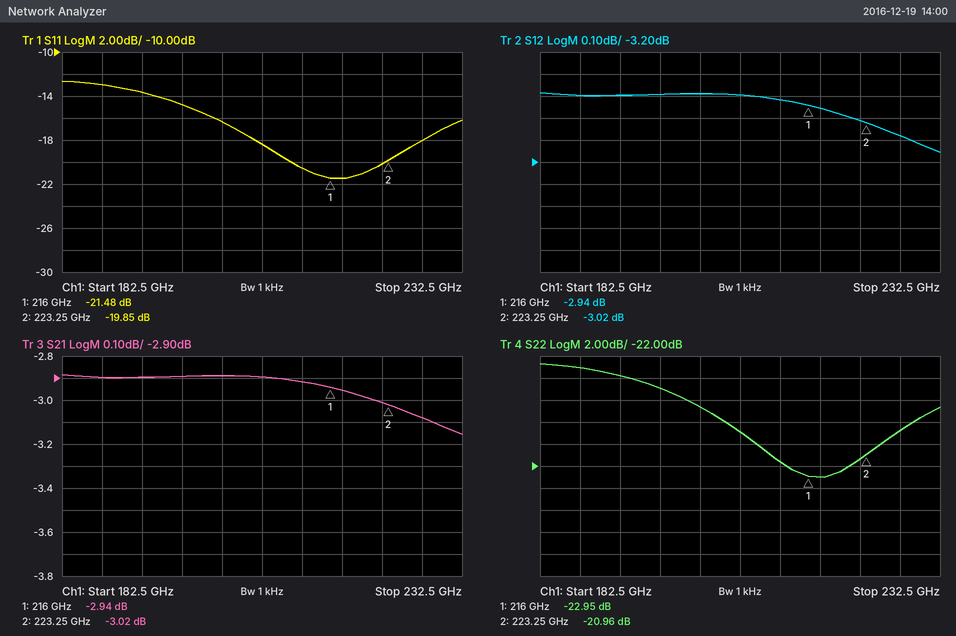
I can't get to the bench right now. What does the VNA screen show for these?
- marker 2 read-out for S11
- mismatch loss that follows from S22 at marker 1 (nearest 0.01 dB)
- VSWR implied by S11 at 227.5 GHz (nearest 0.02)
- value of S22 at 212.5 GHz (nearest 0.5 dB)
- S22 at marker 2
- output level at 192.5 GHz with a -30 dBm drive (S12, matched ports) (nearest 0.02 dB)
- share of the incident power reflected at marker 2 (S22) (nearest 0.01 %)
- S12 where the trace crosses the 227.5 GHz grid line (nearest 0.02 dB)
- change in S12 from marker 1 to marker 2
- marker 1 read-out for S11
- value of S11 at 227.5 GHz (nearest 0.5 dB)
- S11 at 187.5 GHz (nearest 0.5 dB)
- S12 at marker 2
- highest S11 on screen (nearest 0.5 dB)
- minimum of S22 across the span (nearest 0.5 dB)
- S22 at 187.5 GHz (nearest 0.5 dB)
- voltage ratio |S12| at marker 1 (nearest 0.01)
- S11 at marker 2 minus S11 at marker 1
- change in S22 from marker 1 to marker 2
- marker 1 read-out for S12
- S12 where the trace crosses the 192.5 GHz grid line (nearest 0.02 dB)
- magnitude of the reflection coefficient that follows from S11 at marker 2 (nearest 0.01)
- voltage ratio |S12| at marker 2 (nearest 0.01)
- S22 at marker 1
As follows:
-19.85 dB
0.02 dB
1.28
-21.5 dB
-20.96 dB
-32.90 dBm
0.80 %
-3.08 dB
-0.08 dB
-21.48 dB
-18.0 dB
-13.0 dB
-3.02 dB
-12.5 dB
-23.0 dB
-13.0 dB
0.71
1.63 dB
1.99 dB
-2.94 dB
-2.90 dB
0.10
0.71
-22.95 dB
